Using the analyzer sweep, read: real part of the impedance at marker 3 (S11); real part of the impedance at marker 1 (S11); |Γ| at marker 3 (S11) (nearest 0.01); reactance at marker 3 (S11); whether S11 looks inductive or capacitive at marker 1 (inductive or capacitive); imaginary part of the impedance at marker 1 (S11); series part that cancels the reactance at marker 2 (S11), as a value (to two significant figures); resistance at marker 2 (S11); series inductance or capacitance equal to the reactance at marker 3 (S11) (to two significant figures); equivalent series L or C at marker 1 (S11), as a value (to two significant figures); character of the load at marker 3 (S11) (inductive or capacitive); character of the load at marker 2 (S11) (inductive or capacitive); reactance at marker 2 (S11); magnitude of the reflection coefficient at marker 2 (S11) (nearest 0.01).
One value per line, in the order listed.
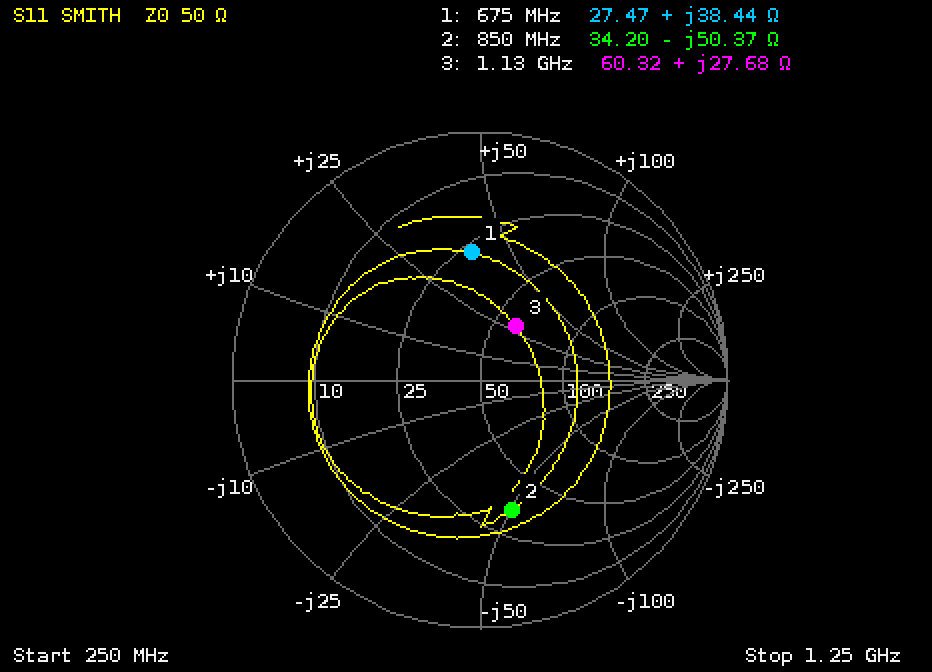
60.32 Ω
27.47 Ω
0.26
+27.68 Ω
inductive
+38.44 Ω
9.4 nH
34.20 Ω
3.9 nH
9.1 nH
inductive
capacitive
-50.37 Ω
0.54
